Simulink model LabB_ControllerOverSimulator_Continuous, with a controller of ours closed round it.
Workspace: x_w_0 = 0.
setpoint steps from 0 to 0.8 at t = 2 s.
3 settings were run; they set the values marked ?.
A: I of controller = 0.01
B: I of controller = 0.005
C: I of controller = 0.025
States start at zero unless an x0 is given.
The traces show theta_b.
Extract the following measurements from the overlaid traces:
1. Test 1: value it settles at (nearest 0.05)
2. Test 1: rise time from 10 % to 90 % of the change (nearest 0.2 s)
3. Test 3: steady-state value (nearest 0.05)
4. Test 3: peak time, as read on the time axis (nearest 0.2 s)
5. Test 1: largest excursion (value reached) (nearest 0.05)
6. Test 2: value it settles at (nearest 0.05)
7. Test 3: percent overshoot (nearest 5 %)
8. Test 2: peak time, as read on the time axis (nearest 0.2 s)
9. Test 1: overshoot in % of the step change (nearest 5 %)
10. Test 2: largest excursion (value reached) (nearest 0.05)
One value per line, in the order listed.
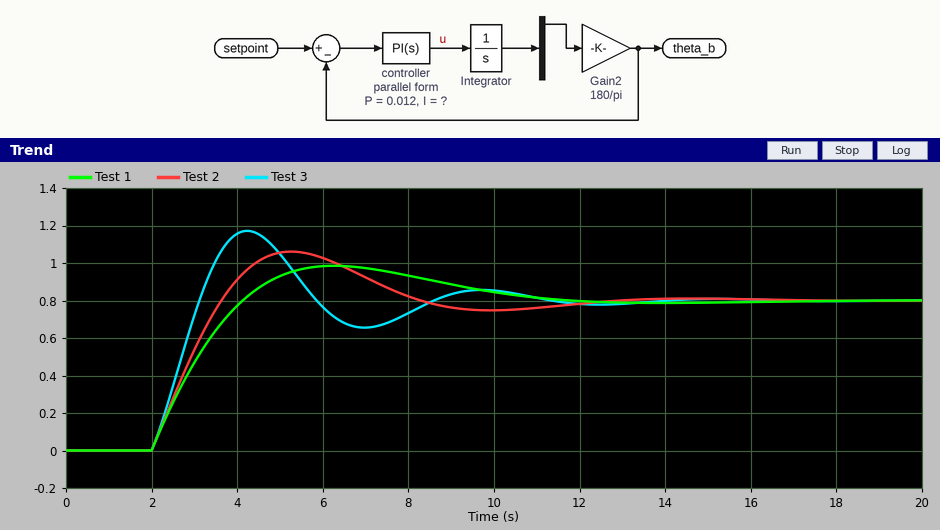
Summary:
0.80
1.6 s
0.80
4.2 s
1.00
0.80
45 %
5.2 s
25 %
1.05
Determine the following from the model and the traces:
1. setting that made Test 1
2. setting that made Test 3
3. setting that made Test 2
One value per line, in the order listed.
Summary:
B
C
A
